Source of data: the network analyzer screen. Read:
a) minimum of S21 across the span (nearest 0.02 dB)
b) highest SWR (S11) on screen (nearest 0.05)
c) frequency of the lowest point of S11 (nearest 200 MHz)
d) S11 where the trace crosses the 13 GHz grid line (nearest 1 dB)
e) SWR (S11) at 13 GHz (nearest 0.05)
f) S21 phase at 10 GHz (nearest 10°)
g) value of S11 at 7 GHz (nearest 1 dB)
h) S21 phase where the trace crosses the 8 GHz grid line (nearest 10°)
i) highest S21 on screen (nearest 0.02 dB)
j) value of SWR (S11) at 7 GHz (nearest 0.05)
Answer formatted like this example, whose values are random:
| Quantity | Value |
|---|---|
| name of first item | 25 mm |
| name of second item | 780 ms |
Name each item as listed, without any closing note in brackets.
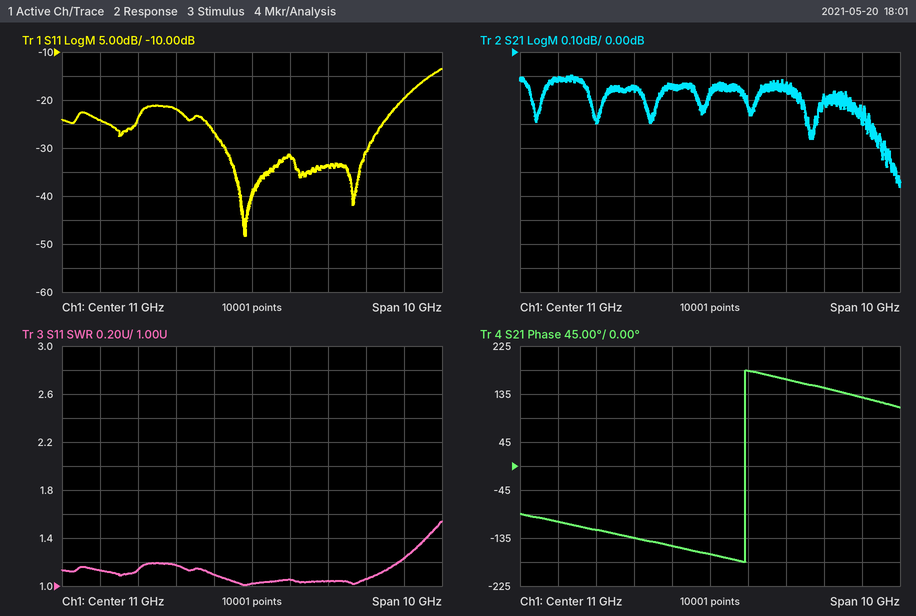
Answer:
| Quantity | Value |
|---|---|
| minimum of S21 across the span | -0.56 dB |
| highest SWR (S11) on screen | 1.55 |
| frequency of the lowest point of S11 | 10.8 GHz |
| S11 where the trace crosses the 13 GHz grid line | -34 dB |
| SWR (S11) at 13 GHz | 1.05 |
| S21 phase at 10 GHz | -150° |
| value of S11 at 7 GHz | -24 dB |
| S21 phase where the trace crosses the 8 GHz grid line | -120° |
| highest S21 on screen | -0.10 dB |
| value of SWR (S11) at 7 GHz | 1.15 |
